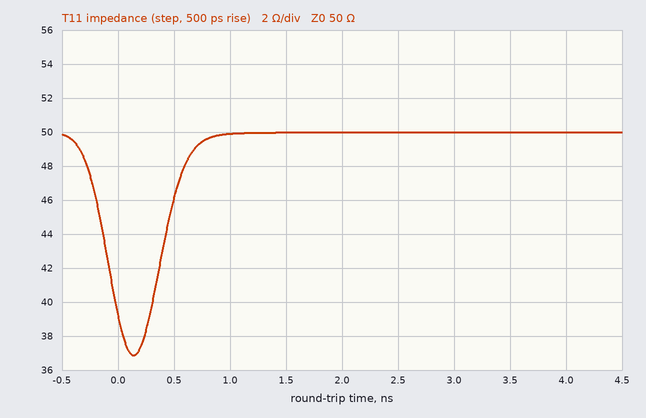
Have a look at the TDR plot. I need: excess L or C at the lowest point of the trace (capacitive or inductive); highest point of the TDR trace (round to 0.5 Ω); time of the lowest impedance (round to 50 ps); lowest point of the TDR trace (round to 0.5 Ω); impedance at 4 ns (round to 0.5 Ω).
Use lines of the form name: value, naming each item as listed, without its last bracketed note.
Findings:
excess L or C at the lowest point of the trace: capacitive
highest point of the TDR trace: 50.0 Ω
time of the lowest impedance: 150 ps
lowest point of the TDR trace: 37.0 Ω
impedance at 4 ns: 50.0 Ω
